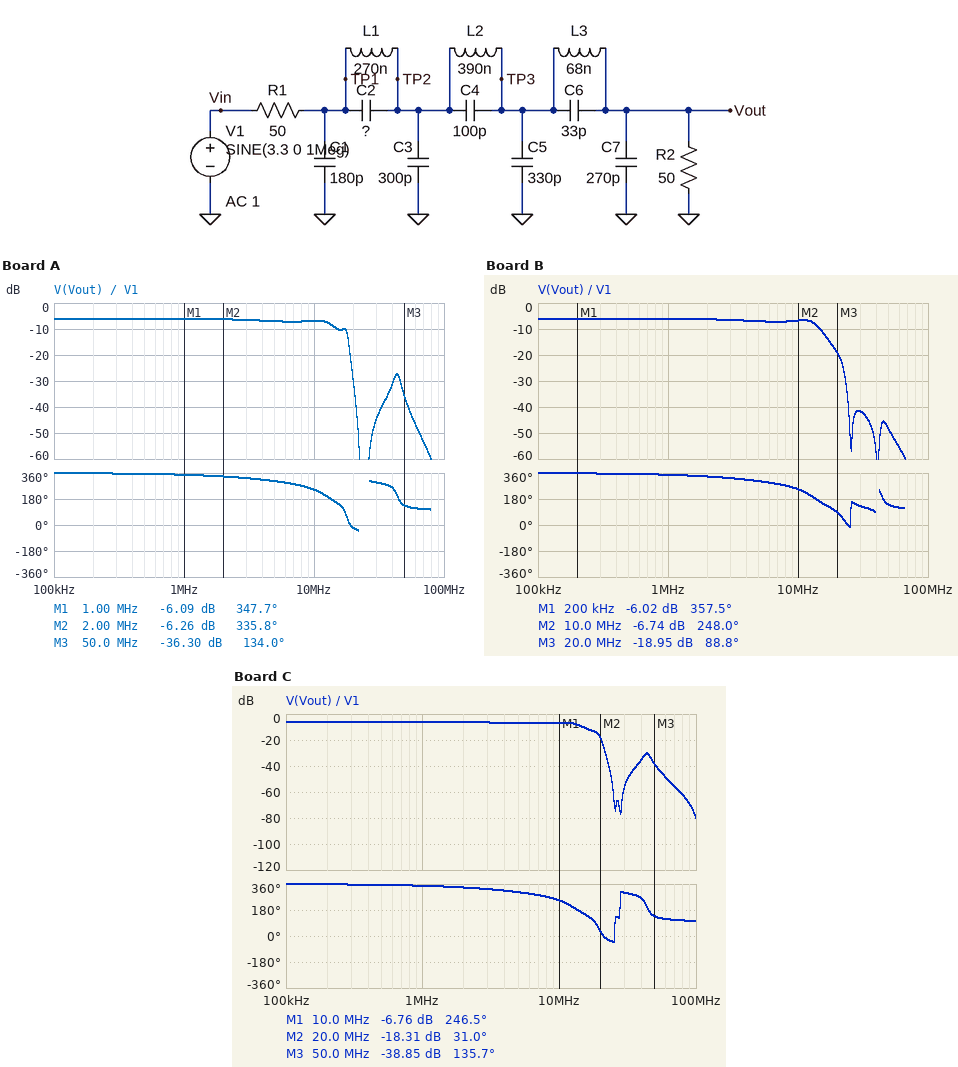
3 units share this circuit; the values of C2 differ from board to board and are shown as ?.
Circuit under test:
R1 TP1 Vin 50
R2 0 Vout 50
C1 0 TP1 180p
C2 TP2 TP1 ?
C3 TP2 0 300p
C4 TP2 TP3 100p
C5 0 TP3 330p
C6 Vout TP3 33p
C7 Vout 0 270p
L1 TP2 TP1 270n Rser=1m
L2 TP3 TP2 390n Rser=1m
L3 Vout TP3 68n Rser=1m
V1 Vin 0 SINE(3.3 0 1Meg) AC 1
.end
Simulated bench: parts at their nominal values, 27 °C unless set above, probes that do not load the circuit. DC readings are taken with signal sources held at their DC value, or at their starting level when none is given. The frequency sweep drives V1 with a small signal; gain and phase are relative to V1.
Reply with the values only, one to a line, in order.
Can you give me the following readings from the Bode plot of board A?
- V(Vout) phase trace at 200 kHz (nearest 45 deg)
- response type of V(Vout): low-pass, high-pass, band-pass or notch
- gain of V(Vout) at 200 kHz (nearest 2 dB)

360 deg
low-pass
-6 dB
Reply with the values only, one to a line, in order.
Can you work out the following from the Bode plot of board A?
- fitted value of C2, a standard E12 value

180 pF
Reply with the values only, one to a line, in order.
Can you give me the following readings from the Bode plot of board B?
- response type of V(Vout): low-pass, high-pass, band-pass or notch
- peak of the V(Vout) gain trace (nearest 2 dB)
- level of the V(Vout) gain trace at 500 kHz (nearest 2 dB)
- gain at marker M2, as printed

low-pass
-6 dB
-6 dB
-6.74 dB
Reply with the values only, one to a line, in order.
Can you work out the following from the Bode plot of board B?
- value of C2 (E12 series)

56 pF
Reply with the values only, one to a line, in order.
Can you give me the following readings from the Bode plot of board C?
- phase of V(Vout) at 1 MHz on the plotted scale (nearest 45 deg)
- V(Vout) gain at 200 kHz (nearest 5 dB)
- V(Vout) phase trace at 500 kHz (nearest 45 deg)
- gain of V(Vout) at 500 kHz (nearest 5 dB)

360 deg
-5 dB
360 deg
-5 dB
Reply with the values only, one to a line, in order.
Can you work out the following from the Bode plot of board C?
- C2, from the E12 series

120 pF
